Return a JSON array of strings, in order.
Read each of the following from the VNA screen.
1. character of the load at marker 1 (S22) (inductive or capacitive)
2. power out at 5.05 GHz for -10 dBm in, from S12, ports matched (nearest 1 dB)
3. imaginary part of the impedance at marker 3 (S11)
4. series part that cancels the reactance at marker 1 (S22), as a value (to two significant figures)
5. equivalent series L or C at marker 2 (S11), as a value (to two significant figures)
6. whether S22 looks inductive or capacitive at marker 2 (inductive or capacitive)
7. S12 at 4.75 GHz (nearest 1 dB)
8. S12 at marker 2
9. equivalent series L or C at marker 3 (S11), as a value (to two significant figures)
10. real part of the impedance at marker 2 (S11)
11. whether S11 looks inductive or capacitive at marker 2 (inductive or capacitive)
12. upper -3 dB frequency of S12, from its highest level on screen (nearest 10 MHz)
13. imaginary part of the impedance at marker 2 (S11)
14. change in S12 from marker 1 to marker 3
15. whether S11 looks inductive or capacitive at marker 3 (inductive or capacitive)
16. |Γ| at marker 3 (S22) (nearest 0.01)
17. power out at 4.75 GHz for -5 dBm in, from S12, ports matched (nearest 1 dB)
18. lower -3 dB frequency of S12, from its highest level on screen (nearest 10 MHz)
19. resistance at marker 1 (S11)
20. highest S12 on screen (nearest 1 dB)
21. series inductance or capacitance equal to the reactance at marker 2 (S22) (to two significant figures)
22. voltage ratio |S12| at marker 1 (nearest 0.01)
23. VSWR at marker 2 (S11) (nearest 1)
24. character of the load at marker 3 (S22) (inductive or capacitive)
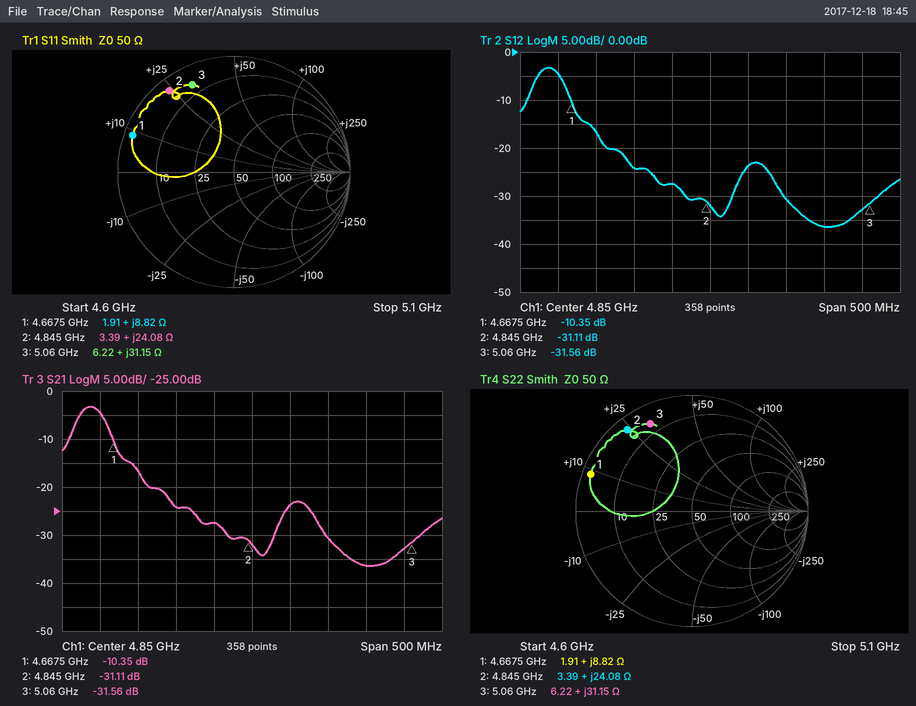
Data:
["inductive", "-43 dBm", "+31.15 Ω", "3.9 pF", "790 pH", "inductive", "-24 dB", "-31.11 dB", "980 pH", "3.39 Ω", "inductive", "4.66 GHz", "+24.08 Ω", "-21.21 dB", "inductive", "0.84", "-29 dBm", "4.62 GHz", "1.91 Ω", "-3 dB", "790 pH", "0.30", "18", "inductive"]
